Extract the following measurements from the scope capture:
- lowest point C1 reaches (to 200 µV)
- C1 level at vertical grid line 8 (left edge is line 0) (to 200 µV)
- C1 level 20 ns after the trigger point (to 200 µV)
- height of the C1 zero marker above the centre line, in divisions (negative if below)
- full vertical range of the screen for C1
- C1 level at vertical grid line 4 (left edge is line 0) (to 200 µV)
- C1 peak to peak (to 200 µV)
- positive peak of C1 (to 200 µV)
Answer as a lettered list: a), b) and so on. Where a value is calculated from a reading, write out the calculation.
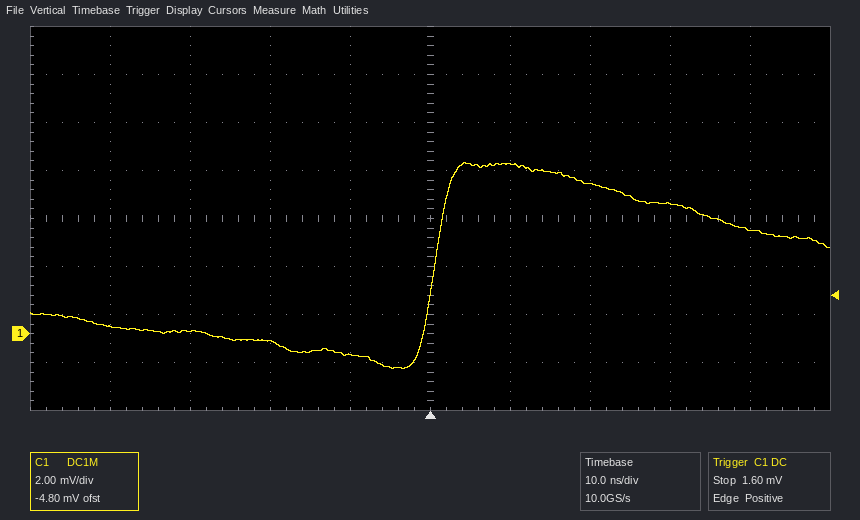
a) -1.4 mV
b) 5.4 mV
c) 6.2 mV
d) -2.4 div
e) 16 mV
f) -800 µV
g) 7.2 mV − (-1.4 mV) = 8.6 mV
h) 7.2 mV
